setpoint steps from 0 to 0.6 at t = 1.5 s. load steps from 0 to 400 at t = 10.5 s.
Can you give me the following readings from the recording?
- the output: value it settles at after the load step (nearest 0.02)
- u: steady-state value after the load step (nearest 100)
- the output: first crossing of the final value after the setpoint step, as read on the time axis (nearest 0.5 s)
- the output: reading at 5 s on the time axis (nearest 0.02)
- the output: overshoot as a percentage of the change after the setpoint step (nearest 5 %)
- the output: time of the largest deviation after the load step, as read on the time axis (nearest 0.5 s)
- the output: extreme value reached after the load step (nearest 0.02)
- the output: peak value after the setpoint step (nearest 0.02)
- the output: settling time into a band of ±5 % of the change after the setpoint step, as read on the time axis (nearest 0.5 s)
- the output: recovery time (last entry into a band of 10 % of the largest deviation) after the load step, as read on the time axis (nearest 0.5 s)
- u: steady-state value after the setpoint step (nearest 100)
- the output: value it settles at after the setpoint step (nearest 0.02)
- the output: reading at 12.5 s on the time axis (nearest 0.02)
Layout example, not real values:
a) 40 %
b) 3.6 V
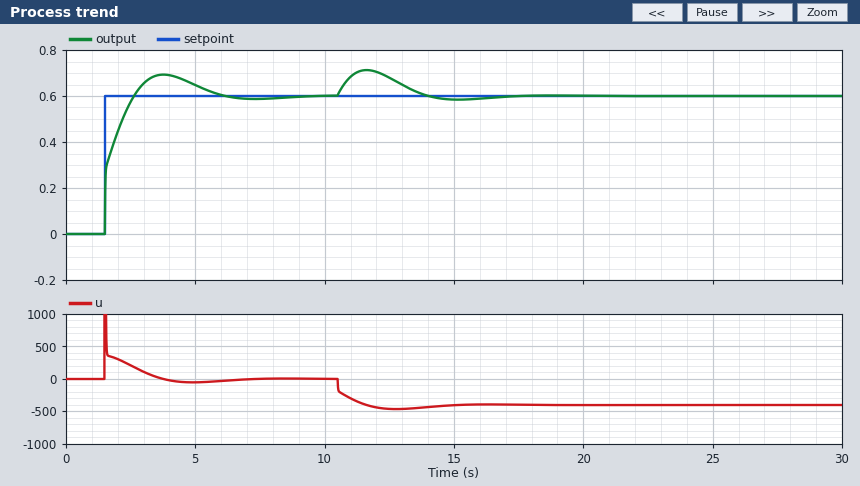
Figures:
a) 0.60
b) -400
c) 2.5 s
d) 0.64
e) 15 %
f) 11.5 s
g) 0.72
h) 0.70
i) 5.5 s
j) 16.0 s
k) 0
l) 0.60
m) 0.68
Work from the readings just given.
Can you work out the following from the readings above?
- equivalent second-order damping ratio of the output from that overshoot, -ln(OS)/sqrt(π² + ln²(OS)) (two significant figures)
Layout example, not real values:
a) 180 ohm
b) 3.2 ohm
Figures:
a) 0.52
